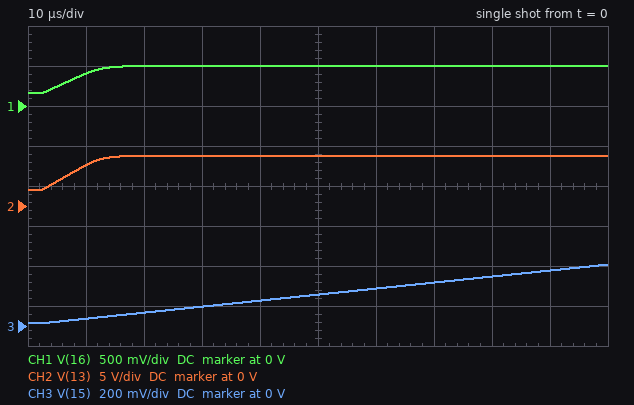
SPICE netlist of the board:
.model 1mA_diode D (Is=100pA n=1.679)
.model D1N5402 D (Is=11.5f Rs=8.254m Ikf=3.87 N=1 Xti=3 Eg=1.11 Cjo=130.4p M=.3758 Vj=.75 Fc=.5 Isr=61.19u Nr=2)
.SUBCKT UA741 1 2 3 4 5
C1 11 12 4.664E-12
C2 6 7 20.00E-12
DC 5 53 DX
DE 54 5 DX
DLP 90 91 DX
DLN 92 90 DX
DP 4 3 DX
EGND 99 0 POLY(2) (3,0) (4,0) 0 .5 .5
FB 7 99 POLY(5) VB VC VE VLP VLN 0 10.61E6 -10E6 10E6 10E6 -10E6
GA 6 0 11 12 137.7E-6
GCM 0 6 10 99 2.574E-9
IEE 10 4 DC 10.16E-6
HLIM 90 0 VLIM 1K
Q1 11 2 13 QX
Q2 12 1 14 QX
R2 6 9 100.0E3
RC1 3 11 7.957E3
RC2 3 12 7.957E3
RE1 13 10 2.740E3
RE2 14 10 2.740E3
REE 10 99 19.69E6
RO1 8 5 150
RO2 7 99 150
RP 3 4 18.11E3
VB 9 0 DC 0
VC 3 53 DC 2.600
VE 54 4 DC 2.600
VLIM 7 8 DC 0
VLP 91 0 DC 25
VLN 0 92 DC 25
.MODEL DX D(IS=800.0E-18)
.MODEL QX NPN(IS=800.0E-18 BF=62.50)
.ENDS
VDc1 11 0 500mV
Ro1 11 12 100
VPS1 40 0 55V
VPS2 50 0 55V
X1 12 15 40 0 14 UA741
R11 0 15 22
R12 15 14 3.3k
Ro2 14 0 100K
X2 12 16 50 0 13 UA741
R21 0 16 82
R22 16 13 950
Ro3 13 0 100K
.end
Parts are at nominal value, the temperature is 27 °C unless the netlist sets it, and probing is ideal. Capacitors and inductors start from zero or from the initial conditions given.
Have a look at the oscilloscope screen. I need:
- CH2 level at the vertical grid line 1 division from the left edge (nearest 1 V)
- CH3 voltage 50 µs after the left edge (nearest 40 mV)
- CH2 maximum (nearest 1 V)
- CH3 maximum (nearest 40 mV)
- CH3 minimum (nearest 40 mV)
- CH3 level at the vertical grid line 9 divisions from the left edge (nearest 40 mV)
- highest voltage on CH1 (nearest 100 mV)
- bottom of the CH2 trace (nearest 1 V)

5 V
160 mV
6 V
320 mV
0 V
280 mV
500 mV
2 V
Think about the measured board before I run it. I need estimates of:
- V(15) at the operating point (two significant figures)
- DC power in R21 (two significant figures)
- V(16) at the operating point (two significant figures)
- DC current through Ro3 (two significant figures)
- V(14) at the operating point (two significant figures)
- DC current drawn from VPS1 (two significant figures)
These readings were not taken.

350 mV
3.1 mW
500 mV
63 µA
53 V
3.0 mA
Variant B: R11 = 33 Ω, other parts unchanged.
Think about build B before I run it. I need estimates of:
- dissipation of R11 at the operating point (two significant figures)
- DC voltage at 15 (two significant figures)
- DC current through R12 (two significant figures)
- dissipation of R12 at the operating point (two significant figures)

7.6 mW
500 mV
15 mA
760 mW
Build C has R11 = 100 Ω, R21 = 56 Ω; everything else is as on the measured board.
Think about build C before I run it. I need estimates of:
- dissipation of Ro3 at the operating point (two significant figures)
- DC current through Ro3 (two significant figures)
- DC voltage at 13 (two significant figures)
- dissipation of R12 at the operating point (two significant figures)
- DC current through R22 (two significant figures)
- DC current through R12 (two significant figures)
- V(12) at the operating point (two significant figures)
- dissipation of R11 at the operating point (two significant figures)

810 µW
90 µA
9.0 V
83 mW
8.9 mA
5.0 mA
500 mV
2.5 mW
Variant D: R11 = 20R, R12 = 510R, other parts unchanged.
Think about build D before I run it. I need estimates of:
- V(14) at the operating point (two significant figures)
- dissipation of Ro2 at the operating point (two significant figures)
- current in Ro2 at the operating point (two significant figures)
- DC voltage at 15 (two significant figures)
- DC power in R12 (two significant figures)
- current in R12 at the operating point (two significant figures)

13 V
1.8 mW
130 µA
500 mV
320 mW
25 mA
